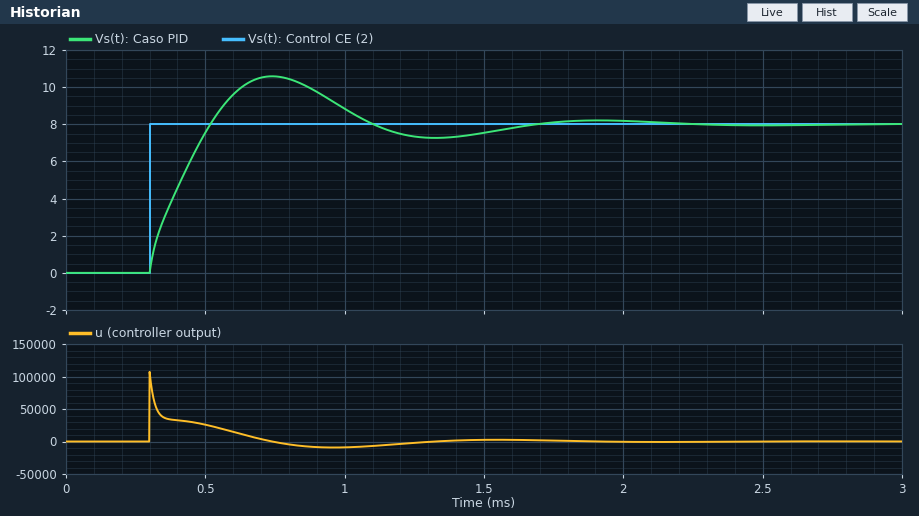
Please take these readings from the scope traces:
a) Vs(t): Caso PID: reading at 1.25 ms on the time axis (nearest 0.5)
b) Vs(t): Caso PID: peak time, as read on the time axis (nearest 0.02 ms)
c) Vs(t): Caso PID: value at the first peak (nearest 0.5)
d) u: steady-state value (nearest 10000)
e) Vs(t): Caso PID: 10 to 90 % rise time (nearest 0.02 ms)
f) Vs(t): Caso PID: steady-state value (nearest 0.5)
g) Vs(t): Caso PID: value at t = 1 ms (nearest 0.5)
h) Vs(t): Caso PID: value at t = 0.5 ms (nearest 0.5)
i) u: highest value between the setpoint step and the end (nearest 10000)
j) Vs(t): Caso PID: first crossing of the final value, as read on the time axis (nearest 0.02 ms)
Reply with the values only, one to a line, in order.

7.5
0.74 ms
10.5
0
0.18 ms
8.0
9.0
7.5
110000
0.52 ms
